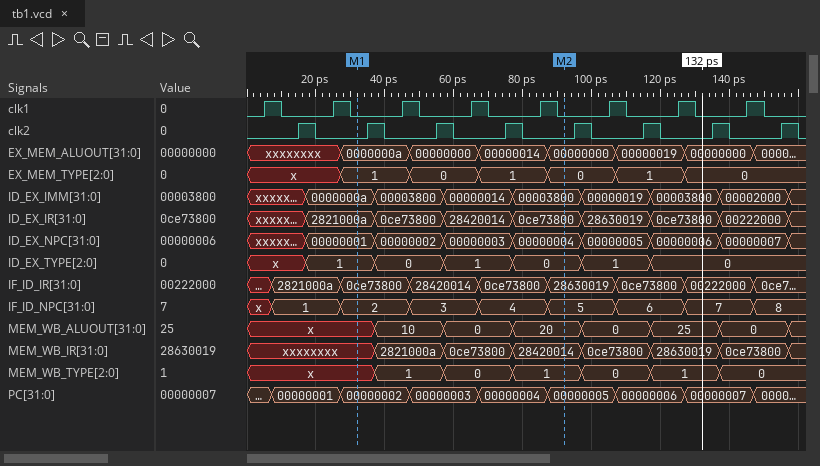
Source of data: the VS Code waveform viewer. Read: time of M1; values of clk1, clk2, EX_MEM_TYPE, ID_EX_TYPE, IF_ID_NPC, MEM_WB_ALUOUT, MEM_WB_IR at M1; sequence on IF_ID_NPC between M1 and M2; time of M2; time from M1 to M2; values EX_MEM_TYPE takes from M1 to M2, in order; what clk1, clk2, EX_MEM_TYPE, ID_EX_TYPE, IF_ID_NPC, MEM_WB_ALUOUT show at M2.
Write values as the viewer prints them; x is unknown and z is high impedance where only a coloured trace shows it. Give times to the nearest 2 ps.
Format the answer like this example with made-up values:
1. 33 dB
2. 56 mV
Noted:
1. 32 ps
2. clk1=0, clk2=0, EX_MEM_TYPE=1, ID_EX_TYPE=1, IF_ID_NPC=2, MEM_WB_ALUOUT=x, MEM_WB_IR=xxxxxxxx
3. 2, 3, 4, 5
4. 92 ps
5. 60 ps
6. 1, 0, 1, 0
7. clk1=0, clk2=0, EX_MEM_TYPE=0, ID_EX_TYPE=0, IF_ID_NPC=5, MEM_WB_ALUOUT=20
